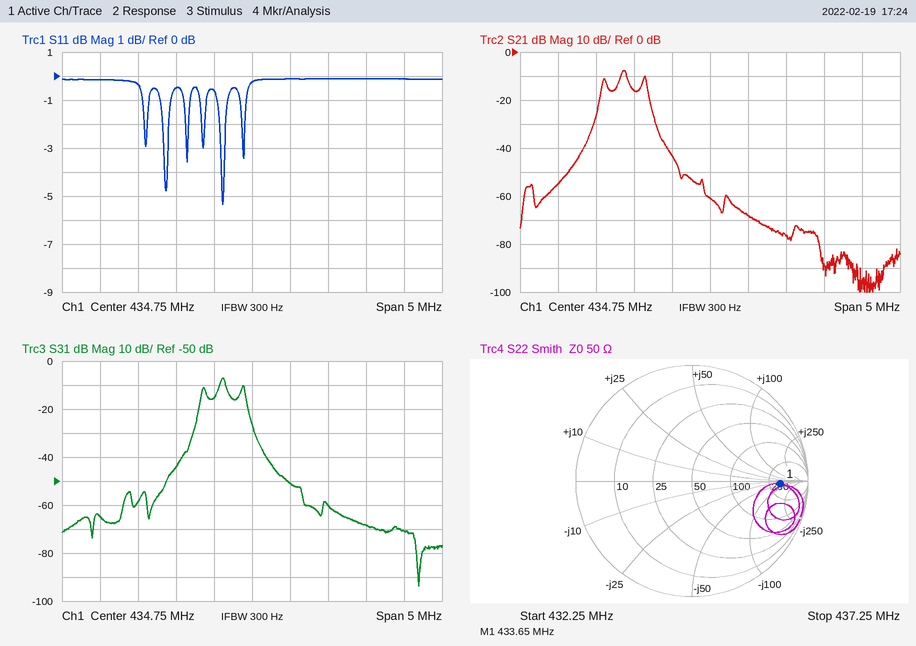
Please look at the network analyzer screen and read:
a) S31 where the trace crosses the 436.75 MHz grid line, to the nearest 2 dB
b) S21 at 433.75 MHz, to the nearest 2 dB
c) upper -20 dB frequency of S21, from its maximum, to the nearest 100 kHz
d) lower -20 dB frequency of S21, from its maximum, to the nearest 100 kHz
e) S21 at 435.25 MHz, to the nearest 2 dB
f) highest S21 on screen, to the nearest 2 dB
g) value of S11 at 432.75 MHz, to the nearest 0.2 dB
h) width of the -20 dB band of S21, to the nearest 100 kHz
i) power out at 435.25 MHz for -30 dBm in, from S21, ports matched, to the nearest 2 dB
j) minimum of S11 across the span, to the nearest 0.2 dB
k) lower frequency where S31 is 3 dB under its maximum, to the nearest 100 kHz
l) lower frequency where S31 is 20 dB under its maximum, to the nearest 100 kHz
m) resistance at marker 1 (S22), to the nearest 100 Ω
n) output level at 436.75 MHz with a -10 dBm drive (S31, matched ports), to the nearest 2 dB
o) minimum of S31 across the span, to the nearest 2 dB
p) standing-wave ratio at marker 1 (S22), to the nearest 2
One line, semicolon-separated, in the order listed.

-70 dB; -16 dB; 434.0 MHz; 433.2 MHz; -68 dB; -8 dB; -0.2 dB; 800 kHz; -98 dBm; -5.4 dB; 434.3 MHz; 434.0 MHz; 400 Ω; -80 dBm; -94 dB; 8
